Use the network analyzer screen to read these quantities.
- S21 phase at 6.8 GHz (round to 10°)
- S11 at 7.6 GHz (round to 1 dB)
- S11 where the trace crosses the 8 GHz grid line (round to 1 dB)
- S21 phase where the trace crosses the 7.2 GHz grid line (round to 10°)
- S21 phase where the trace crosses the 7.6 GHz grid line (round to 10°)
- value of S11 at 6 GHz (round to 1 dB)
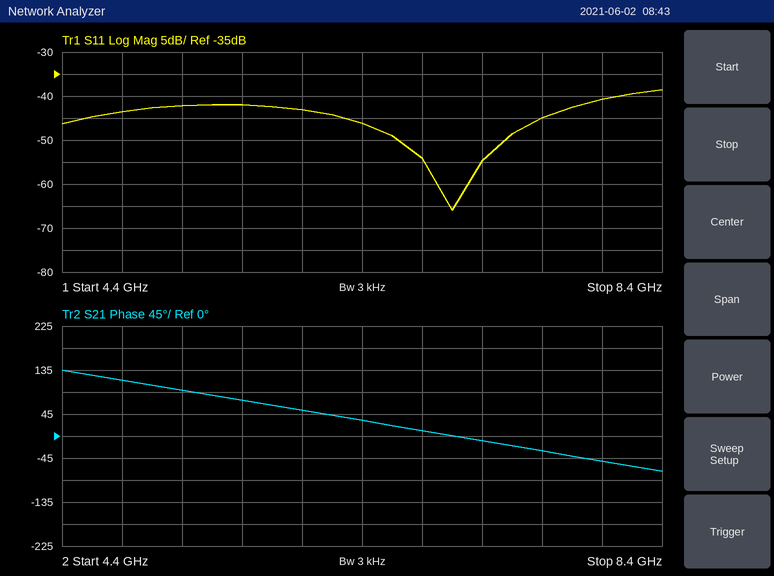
10°
-45 dB
-41 dB
-10°
-30°
-43 dB
